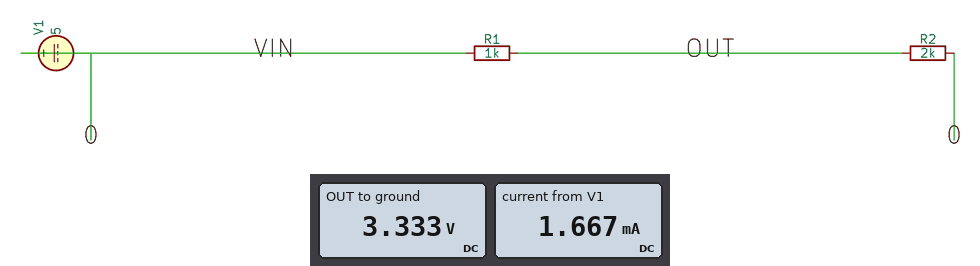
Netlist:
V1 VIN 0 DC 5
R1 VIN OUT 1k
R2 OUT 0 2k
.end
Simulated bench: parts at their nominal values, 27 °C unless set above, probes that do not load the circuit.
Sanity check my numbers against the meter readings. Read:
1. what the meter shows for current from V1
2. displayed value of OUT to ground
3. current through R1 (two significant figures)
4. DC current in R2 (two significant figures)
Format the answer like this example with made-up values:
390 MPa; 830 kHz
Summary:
1.667 mA; 3.333 V; 1.7 mA; 1.7 mA
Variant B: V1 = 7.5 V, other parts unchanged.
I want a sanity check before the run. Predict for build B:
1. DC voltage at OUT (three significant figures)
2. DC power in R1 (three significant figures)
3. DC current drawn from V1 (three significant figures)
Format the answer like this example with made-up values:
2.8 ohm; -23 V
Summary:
5.00 V; 6.25 mW; 2.50 mA
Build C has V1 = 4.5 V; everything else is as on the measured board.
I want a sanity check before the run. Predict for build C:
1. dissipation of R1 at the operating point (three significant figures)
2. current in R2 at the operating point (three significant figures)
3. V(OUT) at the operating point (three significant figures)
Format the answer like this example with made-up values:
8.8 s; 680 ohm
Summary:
2.25 mW; 1.50 mA; 3.00 V
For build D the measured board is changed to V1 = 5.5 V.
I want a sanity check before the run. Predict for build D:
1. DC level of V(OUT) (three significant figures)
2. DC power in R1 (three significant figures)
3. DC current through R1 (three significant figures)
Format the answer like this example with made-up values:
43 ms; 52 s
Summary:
3.67 V; 3.36 mW; 1.83 mA
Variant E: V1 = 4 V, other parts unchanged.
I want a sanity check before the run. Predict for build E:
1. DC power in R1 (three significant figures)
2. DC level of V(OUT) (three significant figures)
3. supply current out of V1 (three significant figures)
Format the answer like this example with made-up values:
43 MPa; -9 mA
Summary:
1.78 mW; 2.67 V; 1.33 mA
